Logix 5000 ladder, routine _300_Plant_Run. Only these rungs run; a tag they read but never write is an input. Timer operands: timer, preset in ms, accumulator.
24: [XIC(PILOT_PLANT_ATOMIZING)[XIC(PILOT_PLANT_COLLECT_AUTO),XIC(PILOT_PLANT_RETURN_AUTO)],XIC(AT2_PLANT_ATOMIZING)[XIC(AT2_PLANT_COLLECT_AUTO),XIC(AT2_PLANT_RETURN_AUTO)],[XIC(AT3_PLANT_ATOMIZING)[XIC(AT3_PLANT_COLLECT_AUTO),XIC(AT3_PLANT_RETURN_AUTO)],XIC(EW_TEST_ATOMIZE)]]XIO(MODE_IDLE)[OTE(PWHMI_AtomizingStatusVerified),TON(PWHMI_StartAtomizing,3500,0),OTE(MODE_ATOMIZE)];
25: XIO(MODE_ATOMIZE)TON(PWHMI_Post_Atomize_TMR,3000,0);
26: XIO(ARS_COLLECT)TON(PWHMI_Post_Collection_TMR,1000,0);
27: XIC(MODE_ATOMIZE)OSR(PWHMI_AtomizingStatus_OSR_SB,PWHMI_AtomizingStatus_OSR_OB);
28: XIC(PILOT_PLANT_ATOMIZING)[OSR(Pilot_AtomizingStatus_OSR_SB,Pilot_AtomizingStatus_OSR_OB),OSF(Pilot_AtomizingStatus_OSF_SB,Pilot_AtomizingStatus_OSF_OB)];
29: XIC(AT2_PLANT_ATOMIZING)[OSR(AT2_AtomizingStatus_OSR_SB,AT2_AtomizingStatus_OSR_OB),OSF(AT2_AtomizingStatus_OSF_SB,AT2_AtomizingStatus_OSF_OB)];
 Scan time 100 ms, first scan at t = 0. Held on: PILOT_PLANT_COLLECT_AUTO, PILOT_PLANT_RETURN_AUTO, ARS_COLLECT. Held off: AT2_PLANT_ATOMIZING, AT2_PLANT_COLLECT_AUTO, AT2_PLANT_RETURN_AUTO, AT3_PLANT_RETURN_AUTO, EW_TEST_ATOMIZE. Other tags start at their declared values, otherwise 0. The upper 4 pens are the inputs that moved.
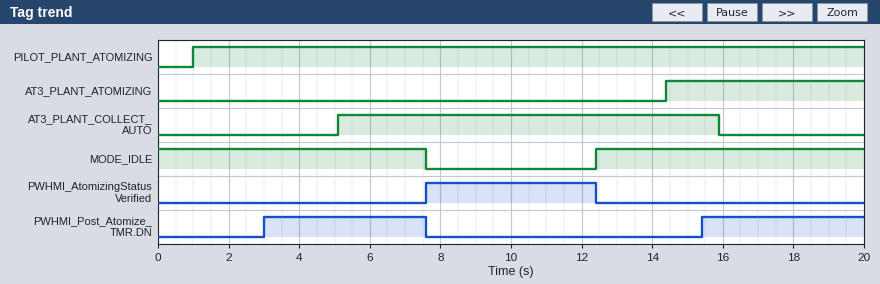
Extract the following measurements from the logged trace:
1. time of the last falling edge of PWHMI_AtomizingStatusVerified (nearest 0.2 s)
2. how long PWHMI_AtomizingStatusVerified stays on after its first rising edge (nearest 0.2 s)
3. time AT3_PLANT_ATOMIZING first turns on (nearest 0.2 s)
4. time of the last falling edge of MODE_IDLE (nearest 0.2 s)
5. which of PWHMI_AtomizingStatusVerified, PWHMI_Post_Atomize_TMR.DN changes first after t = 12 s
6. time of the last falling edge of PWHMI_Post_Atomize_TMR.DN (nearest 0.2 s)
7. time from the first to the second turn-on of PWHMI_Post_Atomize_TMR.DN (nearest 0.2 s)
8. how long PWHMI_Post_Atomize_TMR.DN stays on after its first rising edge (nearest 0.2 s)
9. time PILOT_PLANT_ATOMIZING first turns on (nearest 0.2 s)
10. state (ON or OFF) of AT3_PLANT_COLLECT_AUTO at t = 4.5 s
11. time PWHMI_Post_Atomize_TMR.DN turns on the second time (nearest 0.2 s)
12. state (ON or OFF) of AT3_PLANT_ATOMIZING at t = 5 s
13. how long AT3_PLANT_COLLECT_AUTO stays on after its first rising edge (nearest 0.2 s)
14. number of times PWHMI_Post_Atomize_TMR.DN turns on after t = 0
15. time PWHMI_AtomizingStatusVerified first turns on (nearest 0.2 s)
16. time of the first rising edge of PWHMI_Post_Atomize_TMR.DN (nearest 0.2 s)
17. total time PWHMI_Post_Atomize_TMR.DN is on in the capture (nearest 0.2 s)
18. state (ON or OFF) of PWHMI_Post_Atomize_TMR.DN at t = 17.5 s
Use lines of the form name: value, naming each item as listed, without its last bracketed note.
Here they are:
time of the last falling edge of PWHMI_AtomizingStatusVerified: 12.4 s
how long PWHMI_AtomizingStatusVerified stays on after its first rising edge: 4.8 s
time AT3_PLANT_ATOMIZING first turns on: 14.4 s
time of the last falling edge of MODE_IDLE: 7.6 s
which of PWHMI_AtomizingStatusVerified, PWHMI_Post_Atomize_TMR.DN changes first after t = 12 s: PWHMI_AtomizingStatusVerified
time of the last falling edge of PWHMI_Post_Atomize_TMR.DN: 7.6 s
time from the first to the second turn-on of PWHMI_Post_Atomize_TMR.DN: 12.4 s
how long PWHMI_Post_Atomize_TMR.DN stays on after its first rising edge: 4.6 s
time PILOT_PLANT_ATOMIZING first turns on: 1.0 s
state (ON or OFF) of AT3_PLANT_COLLECT_AUTO at t = 4.5 s: OFF
time PWHMI_Post_Atomize_TMR.DN turns on the second time: 15.4 s
state (ON or OFF) of AT3_PLANT_ATOMIZING at t = 5 s: OFF
how long AT3_PLANT_COLLECT_AUTO stays on after its first rising edge: 10.8 s
number of times PWHMI_Post_Atomize_TMR.DN turns on after t = 0: 2
time PWHMI_AtomizingStatusVerified first turns on: 7.6 s
time of the first rising edge of PWHMI_Post_Atomize_TMR.DN: 3.0 s
total time PWHMI_Post_Atomize_TMR.DN is on in the capture: 9.2 s
state (ON or OFF) of PWHMI_Post_Atomize_TMR.DN at t = 17.5 s: ON
